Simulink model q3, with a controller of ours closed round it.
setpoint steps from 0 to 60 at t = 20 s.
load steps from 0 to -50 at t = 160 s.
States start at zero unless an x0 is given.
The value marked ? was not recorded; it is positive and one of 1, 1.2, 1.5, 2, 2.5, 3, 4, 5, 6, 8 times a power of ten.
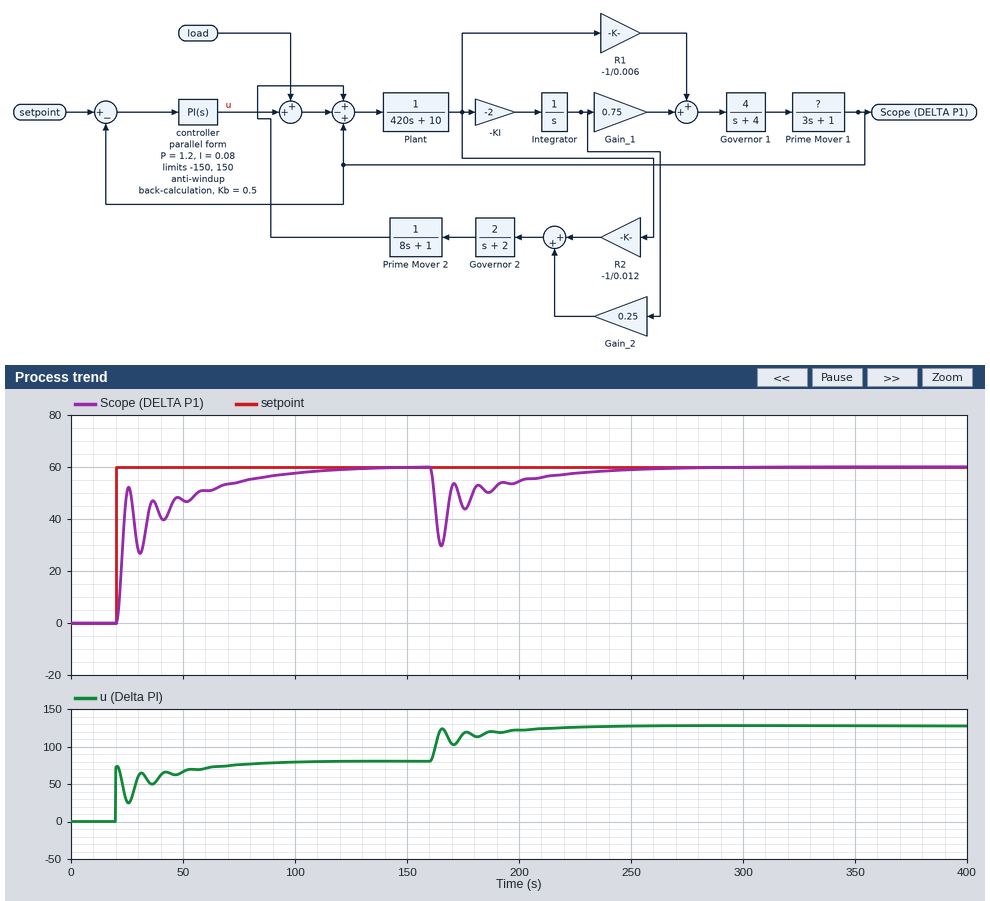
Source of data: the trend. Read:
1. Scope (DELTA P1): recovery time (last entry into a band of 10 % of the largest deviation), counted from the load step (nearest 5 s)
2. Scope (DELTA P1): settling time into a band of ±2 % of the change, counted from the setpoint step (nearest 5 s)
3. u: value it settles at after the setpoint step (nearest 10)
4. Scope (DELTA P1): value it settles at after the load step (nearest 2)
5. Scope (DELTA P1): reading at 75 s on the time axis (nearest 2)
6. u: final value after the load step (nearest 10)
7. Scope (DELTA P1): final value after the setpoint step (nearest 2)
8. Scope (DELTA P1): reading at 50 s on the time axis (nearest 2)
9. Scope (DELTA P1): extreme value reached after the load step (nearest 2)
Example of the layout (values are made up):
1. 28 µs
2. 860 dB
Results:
1. 60 s
2. 95 s
3. 80
4. 60
5. 54
6. 130
7. 60
8. 48
9. 30
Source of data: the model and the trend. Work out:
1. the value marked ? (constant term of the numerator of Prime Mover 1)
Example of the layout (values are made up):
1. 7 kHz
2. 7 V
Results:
1. 1.2
